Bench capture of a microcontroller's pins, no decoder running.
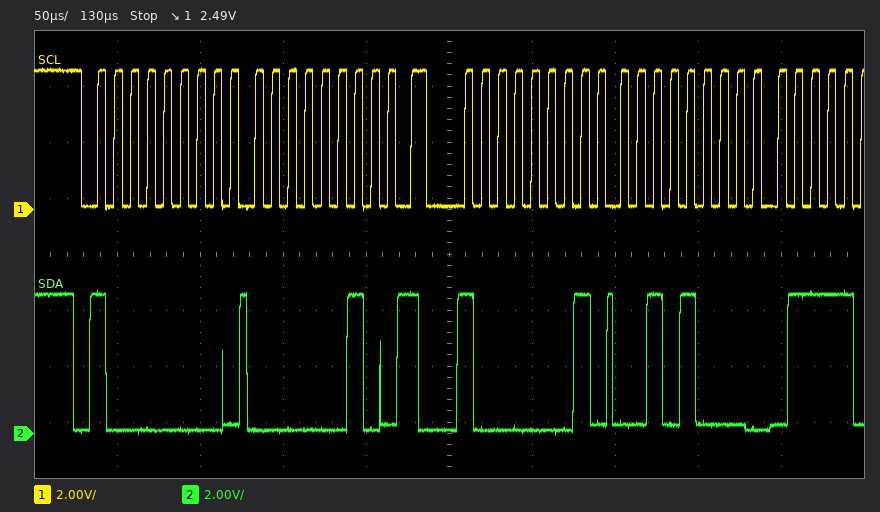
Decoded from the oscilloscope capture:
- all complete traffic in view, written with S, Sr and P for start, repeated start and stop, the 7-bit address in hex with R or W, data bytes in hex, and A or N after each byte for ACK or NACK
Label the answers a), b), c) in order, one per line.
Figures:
a) S 40W A 02 A Sr 40R A 28 A
